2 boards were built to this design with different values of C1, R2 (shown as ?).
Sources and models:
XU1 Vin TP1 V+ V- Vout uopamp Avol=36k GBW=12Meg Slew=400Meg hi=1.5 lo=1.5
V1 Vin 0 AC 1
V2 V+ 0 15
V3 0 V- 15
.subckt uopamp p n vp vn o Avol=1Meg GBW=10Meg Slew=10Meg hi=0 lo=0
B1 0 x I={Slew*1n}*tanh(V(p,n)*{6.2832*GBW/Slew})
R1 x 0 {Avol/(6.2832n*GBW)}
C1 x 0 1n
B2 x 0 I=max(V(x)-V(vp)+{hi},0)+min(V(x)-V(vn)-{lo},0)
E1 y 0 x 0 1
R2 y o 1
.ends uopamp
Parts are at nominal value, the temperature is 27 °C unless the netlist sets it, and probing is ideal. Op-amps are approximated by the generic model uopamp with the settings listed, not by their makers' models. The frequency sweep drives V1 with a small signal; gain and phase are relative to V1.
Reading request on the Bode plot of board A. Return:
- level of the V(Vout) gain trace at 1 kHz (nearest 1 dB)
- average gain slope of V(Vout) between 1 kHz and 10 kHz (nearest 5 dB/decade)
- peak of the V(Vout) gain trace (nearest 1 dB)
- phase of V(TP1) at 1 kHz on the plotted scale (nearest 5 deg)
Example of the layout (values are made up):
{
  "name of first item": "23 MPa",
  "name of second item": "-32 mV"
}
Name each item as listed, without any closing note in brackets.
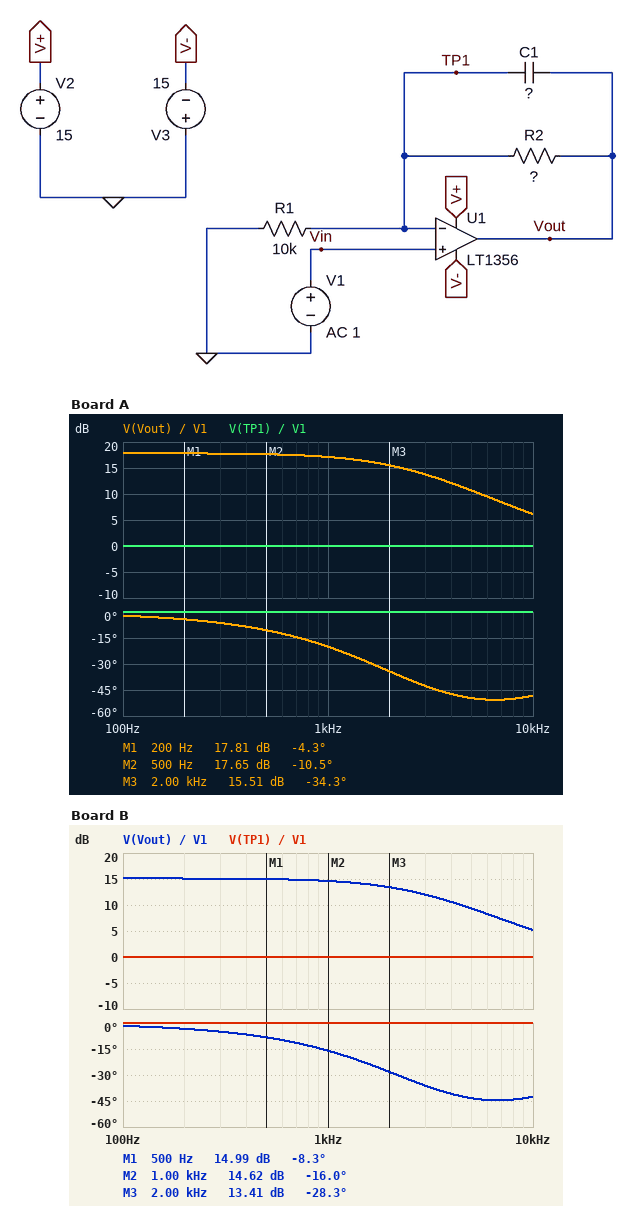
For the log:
{
  "level of the V(Vout) gain trace at 1 kHz": "17 dB",
  "average gain slope of V(Vout) between 1 kHz and 10 kHz": "-10 dB/decade",
  "peak of the V(Vout) gain trace": "18 dB",
  "phase of V(TP1) at 1 kHz on the plotted scale": "0 deg"
}
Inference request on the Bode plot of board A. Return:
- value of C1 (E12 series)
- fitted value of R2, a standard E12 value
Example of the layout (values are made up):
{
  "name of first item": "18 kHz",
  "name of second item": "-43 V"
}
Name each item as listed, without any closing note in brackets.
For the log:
{
  "value of C1": "1 nF",
  "fitted value of R2, a standard E12 value": "68 kΩ"
}
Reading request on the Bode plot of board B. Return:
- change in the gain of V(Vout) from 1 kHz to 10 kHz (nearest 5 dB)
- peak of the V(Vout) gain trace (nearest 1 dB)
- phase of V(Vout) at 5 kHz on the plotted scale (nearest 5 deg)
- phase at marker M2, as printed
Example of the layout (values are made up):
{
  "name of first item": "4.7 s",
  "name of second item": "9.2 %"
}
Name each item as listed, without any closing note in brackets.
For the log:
{
  "change in the gain of V(Vout) from 1 kHz to 10 kHz": "-10 dB",
  "peak of the V(Vout) gain trace": "15 dB",
  "phase of V(Vout) at 5 kHz on the plotted scale": "-45 deg",
  "phase at marker M2, as printed": "-16.0 deg"
}
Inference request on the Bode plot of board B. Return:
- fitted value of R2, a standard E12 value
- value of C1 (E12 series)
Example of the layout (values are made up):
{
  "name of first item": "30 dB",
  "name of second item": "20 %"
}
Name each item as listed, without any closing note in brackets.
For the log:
{
  "fitted value of R2, a standard E12 value": "47 kΩ",
  "value of C1": "1.2 nF"
}
